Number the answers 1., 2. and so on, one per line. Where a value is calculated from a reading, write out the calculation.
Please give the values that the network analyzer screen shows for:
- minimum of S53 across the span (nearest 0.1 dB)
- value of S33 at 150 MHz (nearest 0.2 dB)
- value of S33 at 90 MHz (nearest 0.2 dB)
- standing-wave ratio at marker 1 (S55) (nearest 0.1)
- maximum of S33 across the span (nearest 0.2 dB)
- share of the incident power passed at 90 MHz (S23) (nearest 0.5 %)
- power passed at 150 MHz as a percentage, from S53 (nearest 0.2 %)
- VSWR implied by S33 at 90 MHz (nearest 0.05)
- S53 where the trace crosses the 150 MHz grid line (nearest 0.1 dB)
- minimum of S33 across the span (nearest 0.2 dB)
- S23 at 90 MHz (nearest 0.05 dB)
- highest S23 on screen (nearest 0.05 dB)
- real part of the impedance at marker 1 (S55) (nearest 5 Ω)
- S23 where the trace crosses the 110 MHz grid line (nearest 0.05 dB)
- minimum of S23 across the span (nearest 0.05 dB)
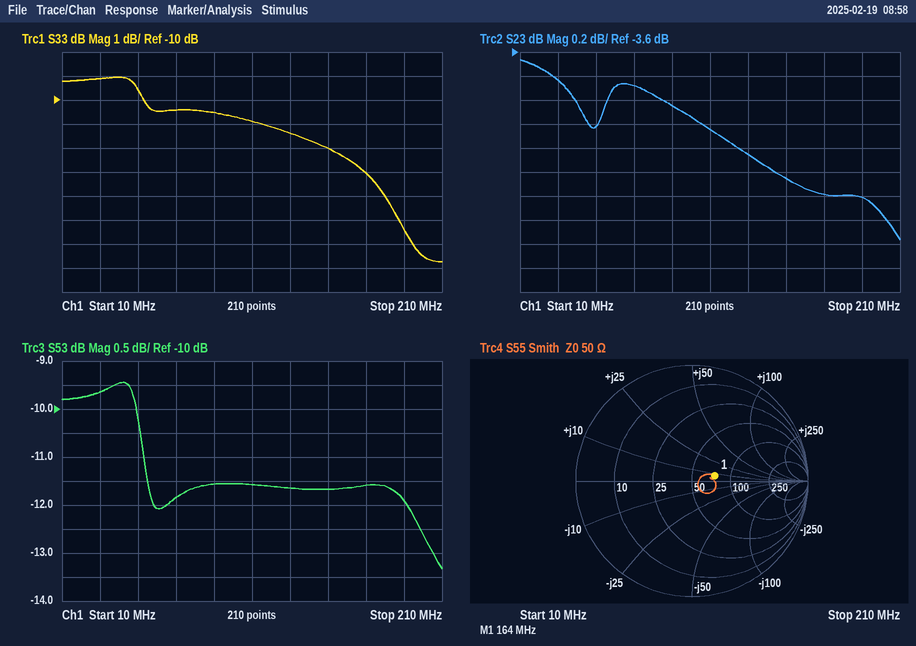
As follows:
1. -13.3 dB
2. -12.0 dB
3. -10.6 dB
4. 1.5
5. -9.0 dB
6. 10^(-4.05/10) ≈ 39.4 %, so 39.5 % to the nearest 0.5 %
7. 10^(-11.7/10) ≈ 6.8 %
8. |Γ| = 10^(-10.6/20) = 0.2951; VSWR = (1 + 0.2951)/(1 − 0.2951) ≈ 1.84, so 1.85 to the nearest 0.05
9. -11.7 dB
10. -16.8 dB
11. -4.05 dB
12. -3.65 dB
13. 75 Ω
14. -4.25 dB
15. -5.15 dB
